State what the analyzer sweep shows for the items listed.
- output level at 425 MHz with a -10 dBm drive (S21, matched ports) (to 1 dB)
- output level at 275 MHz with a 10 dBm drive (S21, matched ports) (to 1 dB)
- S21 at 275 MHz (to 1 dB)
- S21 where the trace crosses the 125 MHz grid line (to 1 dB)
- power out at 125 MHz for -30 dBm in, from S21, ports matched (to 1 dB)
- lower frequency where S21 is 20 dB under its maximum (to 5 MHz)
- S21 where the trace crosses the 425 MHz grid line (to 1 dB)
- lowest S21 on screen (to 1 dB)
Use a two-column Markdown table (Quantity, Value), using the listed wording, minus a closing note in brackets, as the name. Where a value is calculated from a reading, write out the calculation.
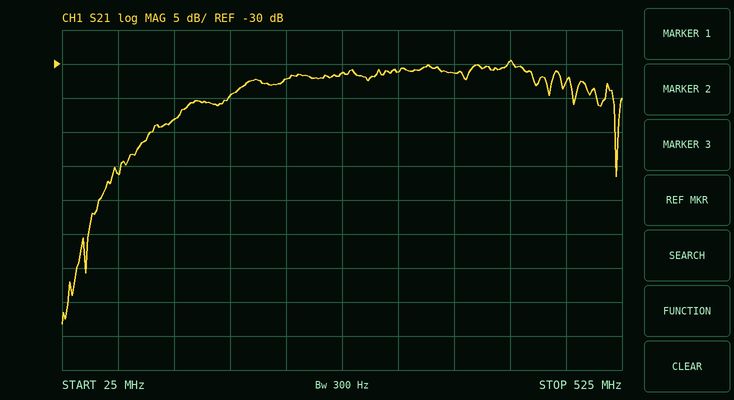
| Quantity | Value |
|---|---|
| output level at 425 MHz with a -10 dBm drive (S21, matched ports) | -10 dBm + (-30 dB) = -40 dBm |
| output level at 275 MHz with a 10 dBm drive (S21, matched ports) | 10 dBm + (-31 dB) = -21 dBm |
| S21 at 275 MHz | -31 dB |
| S21 where the trace crosses the 125 MHz grid line | -38 dB |
| power out at 125 MHz for -30 dBm in, from S21, ports matched | -30 dBm + (-38 dB) = -68 dBm |
| lower frequency where S21 is 20 dB under its maximum | 60 MHz |
| S21 where the trace crosses the 425 MHz grid line | -30 dB |
| lowest S21 on screen | -68 dB |
